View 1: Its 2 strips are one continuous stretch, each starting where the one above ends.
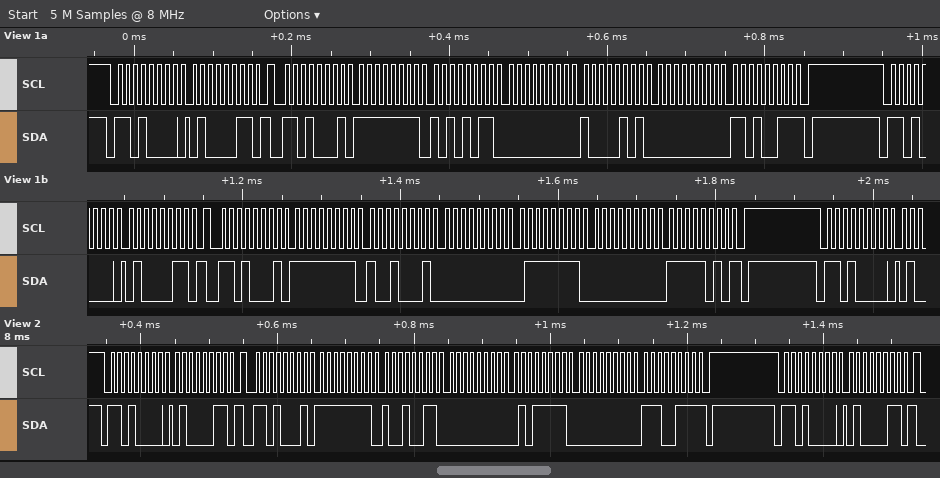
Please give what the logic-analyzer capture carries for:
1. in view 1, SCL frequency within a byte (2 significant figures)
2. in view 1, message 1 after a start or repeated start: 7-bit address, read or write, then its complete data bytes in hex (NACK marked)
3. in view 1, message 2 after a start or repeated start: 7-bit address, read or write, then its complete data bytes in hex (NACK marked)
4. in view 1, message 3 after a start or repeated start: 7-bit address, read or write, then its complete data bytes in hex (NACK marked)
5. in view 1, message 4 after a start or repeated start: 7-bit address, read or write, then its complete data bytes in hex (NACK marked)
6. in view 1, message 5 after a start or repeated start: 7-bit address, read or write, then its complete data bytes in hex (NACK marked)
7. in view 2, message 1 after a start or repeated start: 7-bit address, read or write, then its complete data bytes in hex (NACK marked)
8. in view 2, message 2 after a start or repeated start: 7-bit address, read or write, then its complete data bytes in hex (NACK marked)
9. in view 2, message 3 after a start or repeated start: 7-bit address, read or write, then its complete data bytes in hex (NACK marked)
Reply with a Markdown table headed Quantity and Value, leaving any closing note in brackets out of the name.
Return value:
| Quantity | Value |
|---|---|
| in view 1, SCL frequency within a byte | 100 kHz |
| in view 1, message 1 after a start or repeated start: 7-bit address, read or write, then its complete data bytes in hex | 0x68 write: 43 |
| in view 1, message 2 after a start or repeated start: 7-bit address, read or write, then its complete data bytes in hex | 0x68 read: FF AB 00 85 00 D3 NACK |
| in view 1, message 3 after a start or repeated start: 7-bit address, read or write, then its complete data bytes in hex | 0x68 write: 43 |
| in view 1, message 4 after a start or repeated start: 7-bit address, read or write, then its complete data bytes in hex | 0x68 read: FF 91 00 7F 00 FA NACK |
| in view 1, message 5 after a start or repeated start: 7-bit address, read or write, then its complete data bytes in hex | 0x68 write |
| in view 2, message 1 after a start or repeated start: 7-bit address, read or write, then its complete data bytes in hex | 0x68 write: 43 |
| in view 2, message 2 after a start or repeated start: 7-bit address, read or write, then its complete data bytes in hex | 0x68 read: FF 93 00 5F 00 E7 NACK |
| in view 2, message 3 after a start or repeated start: 7-bit address, read or write, then its complete data bytes in hex | 0x68 write: 43 |
